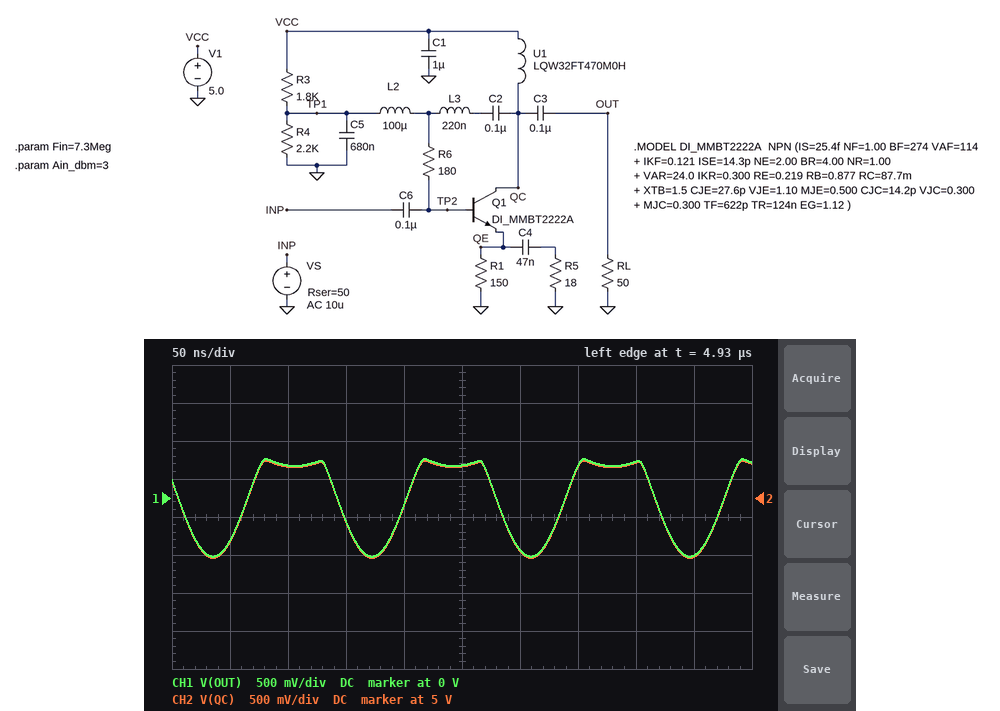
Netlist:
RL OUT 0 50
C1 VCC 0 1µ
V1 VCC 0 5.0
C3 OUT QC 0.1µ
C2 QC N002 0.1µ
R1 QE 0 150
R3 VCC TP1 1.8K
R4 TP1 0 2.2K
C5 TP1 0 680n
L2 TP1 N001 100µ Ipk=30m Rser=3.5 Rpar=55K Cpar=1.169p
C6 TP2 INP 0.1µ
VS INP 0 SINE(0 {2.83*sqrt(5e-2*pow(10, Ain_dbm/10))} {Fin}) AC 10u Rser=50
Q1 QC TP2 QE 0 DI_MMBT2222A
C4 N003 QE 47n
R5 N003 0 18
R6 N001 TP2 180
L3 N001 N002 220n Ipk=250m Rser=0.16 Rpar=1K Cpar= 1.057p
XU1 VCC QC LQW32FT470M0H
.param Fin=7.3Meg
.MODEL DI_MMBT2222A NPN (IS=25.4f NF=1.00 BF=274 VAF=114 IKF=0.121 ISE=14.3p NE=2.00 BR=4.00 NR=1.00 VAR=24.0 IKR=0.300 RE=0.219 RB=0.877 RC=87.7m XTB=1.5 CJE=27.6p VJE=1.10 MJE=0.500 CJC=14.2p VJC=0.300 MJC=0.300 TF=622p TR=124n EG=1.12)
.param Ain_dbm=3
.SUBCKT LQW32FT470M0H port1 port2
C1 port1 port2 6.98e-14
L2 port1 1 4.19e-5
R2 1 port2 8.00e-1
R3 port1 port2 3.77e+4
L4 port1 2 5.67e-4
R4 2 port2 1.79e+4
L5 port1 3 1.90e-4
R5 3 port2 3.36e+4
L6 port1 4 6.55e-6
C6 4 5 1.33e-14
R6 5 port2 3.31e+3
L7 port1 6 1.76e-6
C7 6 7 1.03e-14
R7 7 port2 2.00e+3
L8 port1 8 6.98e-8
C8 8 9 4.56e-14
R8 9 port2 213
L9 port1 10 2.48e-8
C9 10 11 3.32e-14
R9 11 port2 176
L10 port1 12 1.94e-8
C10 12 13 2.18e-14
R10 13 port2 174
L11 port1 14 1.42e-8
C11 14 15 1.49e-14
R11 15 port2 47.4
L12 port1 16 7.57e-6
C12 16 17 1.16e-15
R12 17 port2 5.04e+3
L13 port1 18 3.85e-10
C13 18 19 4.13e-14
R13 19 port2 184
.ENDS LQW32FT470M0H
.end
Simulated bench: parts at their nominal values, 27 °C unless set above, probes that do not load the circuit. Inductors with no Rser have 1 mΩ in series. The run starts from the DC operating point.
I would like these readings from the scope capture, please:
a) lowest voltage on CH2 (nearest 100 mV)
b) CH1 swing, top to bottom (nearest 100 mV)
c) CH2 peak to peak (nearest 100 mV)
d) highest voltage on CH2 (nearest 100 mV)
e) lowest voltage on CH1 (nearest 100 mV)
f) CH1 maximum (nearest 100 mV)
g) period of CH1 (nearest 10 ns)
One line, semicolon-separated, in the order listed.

4.2 V; 1.3 V; 1.3 V; 5.5 V; -800 mV; 500 mV; 140 ns
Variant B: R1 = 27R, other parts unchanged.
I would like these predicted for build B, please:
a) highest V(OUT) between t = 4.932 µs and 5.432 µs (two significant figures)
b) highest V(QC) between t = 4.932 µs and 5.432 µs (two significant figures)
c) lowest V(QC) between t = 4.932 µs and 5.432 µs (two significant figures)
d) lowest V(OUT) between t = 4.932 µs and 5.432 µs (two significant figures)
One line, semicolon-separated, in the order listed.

1.3 V; 6.2 V; 3.7 V; -1.3 V
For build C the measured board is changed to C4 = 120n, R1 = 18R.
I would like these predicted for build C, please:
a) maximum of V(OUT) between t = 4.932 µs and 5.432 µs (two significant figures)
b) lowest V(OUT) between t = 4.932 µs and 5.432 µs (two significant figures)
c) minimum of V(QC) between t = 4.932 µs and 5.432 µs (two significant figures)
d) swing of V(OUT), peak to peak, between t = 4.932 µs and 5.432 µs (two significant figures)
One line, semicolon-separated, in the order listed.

1.4 V; -1.4 V; 3.5 V; 2.8 V
